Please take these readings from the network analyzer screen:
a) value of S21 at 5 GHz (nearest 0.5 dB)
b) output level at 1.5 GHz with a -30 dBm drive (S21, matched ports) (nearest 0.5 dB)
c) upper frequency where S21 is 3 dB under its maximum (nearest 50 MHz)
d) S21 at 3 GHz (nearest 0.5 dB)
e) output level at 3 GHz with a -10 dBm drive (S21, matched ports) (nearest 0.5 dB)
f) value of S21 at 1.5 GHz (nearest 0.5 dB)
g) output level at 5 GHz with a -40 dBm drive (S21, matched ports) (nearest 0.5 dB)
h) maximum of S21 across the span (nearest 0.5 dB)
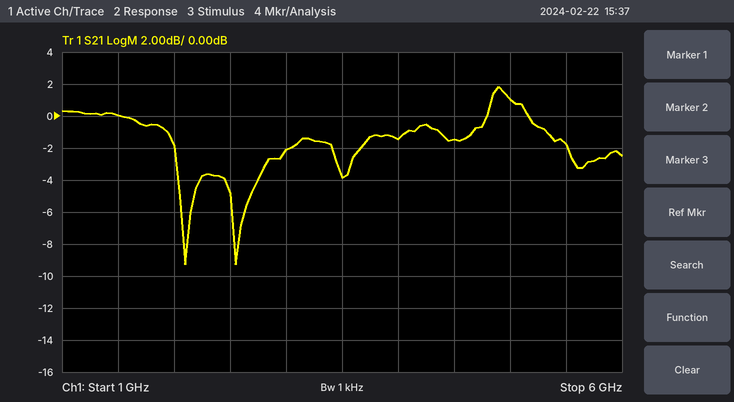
1.0 dB
-30.0 dBm
5.35 GHz
-2.0 dB
-12.0 dBm
0.0 dB
-39.0 dBm
2.0 dB
